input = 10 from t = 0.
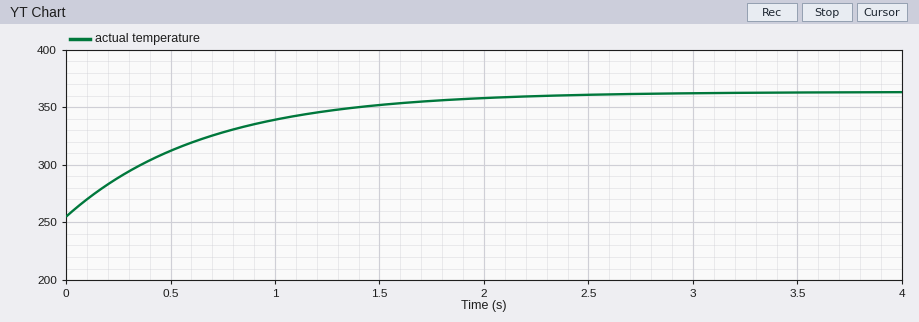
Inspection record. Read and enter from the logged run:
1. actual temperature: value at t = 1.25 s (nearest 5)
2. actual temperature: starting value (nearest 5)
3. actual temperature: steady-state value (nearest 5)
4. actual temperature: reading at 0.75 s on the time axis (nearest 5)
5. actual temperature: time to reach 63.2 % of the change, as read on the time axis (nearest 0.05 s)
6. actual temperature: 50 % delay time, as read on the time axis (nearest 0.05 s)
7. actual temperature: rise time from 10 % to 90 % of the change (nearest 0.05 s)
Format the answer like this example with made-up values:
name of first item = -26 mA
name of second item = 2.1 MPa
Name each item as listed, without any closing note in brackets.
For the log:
actual temperature: value at t = 1.25 s = 345
actual temperature: starting value = 255
actual temperature: steady-state value = 365
actual temperature: reading at 0.75 s on the time axis = 330
actual temperature: time to reach 63.2 % of the change, as read on the time axis = 0.65 s
actual temperature: 50 % delay time, as read on the time axis = 0.45 s
actual temperature: rise time from 10 % to 90 % of the change = 1.45 s
